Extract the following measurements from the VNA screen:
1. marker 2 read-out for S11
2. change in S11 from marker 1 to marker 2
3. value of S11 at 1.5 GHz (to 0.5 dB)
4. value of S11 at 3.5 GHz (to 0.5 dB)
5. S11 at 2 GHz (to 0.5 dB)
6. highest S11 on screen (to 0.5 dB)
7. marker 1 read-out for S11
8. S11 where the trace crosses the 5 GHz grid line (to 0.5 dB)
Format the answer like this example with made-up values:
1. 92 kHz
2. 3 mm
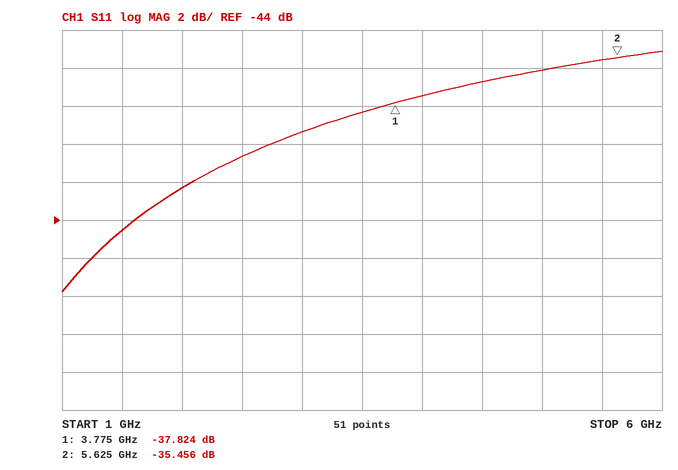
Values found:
1. -35.456 dB
2. 2.368 dB
3. -44.5 dB
4. -38.5 dB
5. -42.5 dB
6. -35.0 dB
7. -37.824 dB
8. -36.0 dB
